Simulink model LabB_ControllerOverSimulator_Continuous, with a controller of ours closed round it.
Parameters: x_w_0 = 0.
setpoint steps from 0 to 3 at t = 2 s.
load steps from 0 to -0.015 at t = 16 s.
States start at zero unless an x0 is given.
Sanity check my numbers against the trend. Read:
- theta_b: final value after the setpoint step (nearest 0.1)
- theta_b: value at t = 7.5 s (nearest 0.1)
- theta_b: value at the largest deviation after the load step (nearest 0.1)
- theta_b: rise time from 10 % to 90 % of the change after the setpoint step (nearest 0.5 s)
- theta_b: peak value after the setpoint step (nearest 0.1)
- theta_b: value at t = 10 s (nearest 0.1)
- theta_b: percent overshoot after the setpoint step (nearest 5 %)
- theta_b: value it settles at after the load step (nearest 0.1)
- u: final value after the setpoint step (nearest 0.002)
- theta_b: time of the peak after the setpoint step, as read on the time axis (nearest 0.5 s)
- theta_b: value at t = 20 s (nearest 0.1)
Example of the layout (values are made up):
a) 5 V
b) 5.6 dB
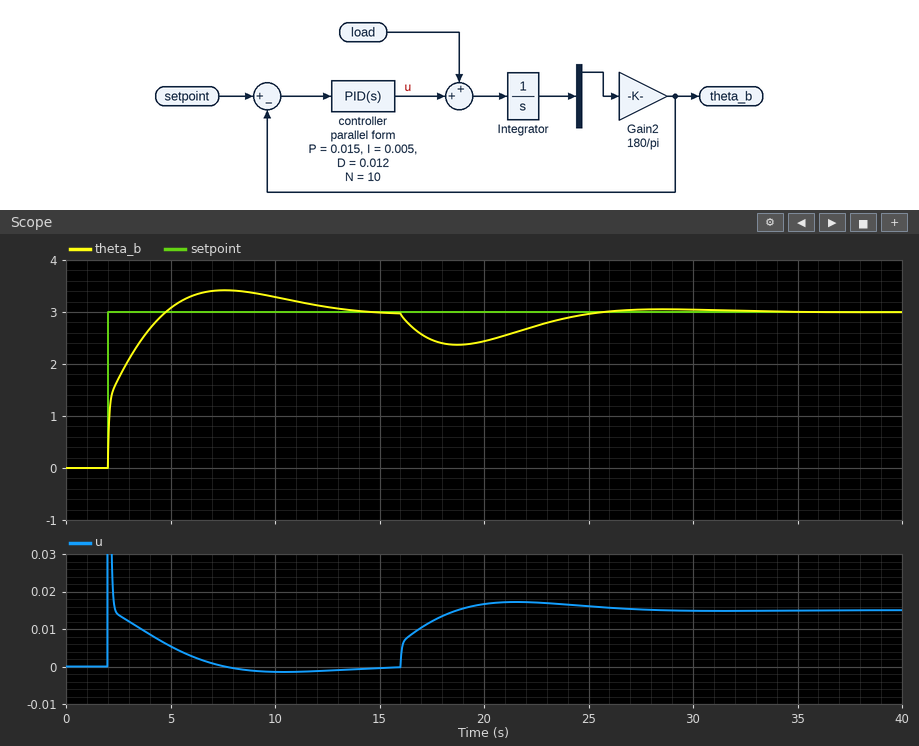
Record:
a) 3.0
b) 3.4
c) 2.4
d) 2.0 s
e) 3.4
f) 3.3
g) 15 %
h) 3.0
i) 0.000
j) 7.5 s
k) 2.4
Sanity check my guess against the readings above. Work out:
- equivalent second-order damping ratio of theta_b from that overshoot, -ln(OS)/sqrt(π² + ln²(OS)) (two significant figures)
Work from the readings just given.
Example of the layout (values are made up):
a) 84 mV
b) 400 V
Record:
a) 0.52
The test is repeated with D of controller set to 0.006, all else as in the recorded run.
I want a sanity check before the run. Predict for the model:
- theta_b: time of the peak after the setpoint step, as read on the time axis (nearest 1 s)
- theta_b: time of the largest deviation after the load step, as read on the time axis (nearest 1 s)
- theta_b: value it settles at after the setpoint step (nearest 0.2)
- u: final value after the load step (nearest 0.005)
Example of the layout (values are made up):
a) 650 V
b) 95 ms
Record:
a) 7 s
b) 18 s
c) 3.0
d) 0.015
